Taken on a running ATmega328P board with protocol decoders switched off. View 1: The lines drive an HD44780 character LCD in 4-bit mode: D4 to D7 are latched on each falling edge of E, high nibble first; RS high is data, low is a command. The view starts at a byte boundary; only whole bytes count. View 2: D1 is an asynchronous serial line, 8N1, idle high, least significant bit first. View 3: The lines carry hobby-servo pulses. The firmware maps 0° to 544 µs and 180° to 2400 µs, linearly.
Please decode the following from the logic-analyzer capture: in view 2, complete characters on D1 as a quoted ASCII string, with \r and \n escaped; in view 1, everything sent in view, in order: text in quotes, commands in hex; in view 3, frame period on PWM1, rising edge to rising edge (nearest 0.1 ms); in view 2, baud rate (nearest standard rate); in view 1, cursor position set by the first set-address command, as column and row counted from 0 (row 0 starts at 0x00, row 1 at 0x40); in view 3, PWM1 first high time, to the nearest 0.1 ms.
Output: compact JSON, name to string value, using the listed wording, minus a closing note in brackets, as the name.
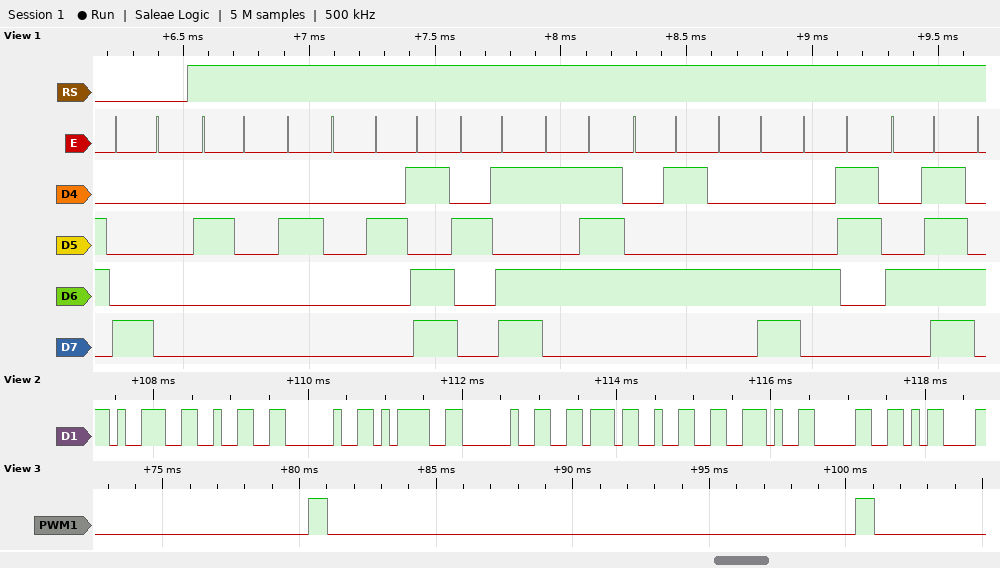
{"in view 2, complete characters on D1 as a quoted ASCII string, with \\r and \\n escaped": "\"92 = v2.0\\r\"", "in view 1, everything sent in view, in order: text in quotes, commands in hex": "0x80 \"  --WELCO\"", "in view 3, frame period on PWM1, rising edge to rising edge": "20.0 ms", "in view 2, baud rate": "9600 baud", "in view 1, cursor position set by the first set-address command, as column and row counted from 0": "column 0, row 0", "in view 3, PWM1 first high time, to the nearest 0.1 ms": "0.7 ms"}
